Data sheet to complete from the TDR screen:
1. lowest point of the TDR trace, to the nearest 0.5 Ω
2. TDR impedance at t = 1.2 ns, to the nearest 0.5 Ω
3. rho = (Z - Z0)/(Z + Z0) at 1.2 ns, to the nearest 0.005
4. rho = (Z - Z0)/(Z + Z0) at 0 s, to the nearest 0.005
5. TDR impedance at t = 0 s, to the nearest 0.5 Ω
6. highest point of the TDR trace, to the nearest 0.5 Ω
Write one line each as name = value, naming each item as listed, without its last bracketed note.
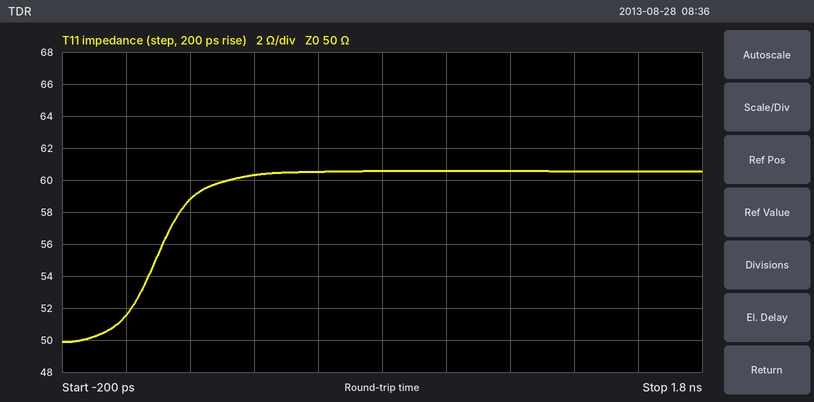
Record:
lowest point of the TDR trace, to the nearest 0.5 Ω = 50.0 Ω
TDR impedance at t = 1.2 ns, to the nearest 0.5 Ω = 60.5 Ω
rho = (Z - Z0)/(Z + Z0) at 1.2 ns, to the nearest 0.005 = +0.095
rho = (Z - Z0)/(Z + Z0) at 0 s, to the nearest 0.005 = +0.015
TDR impedance at t = 0 s, to the nearest 0.5 Ω = 51.5 Ω
highest point of the TDR trace, to the nearest 0.5 Ω = 60.5 Ω
